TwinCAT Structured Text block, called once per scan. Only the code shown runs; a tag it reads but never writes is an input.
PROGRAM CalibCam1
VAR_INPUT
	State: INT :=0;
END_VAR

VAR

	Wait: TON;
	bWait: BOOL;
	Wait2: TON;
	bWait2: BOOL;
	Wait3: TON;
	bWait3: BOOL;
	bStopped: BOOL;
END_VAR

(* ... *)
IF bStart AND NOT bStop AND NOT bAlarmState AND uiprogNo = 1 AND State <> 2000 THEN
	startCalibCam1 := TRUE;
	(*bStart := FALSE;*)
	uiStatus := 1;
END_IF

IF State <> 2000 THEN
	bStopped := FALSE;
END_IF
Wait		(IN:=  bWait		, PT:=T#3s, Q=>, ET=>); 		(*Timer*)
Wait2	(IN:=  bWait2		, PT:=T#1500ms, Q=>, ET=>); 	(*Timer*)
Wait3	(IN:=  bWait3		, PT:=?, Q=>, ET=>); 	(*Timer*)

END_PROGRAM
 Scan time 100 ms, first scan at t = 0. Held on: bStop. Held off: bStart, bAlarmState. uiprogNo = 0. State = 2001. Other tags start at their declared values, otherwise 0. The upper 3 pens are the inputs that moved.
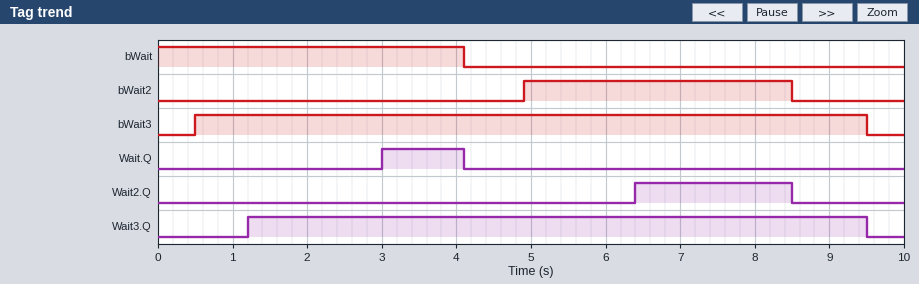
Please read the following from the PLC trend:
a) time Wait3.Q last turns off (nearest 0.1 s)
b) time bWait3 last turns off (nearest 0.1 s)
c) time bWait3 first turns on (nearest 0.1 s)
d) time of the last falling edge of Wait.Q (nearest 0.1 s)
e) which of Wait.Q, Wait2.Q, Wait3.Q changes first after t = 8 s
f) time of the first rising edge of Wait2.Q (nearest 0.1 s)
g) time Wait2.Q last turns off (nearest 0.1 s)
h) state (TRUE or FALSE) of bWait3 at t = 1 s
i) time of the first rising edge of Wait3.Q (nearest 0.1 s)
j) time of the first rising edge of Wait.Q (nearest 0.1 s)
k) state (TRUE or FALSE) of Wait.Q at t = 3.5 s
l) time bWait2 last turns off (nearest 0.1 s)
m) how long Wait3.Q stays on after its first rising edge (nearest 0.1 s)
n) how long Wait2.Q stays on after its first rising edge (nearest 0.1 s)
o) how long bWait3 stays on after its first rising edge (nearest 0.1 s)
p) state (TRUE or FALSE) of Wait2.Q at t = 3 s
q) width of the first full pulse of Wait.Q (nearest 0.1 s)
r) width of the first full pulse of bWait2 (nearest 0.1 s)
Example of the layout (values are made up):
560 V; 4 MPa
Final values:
9.5 s; 9.5 s; 0.5 s; 4.1 s; Wait2.Q; 6.4 s; 8.5 s; TRUE; 1.2 s; 3.0 s; TRUE; 8.5 s; 8.3 s; 2.1 s; 9.0 s; FALSE; 1.1 s; 3.6 s
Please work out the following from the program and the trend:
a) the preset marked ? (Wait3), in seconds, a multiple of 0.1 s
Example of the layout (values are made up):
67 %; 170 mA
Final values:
0.7 s
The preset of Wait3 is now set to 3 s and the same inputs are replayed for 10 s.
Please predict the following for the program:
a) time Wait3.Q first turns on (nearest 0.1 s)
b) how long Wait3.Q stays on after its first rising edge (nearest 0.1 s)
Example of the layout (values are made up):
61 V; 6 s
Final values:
3.5 s; 6.0 s
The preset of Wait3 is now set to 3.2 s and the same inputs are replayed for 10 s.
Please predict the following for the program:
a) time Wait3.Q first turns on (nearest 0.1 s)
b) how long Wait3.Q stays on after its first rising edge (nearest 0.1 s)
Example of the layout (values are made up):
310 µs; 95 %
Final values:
3.7 s; 5.8 s
